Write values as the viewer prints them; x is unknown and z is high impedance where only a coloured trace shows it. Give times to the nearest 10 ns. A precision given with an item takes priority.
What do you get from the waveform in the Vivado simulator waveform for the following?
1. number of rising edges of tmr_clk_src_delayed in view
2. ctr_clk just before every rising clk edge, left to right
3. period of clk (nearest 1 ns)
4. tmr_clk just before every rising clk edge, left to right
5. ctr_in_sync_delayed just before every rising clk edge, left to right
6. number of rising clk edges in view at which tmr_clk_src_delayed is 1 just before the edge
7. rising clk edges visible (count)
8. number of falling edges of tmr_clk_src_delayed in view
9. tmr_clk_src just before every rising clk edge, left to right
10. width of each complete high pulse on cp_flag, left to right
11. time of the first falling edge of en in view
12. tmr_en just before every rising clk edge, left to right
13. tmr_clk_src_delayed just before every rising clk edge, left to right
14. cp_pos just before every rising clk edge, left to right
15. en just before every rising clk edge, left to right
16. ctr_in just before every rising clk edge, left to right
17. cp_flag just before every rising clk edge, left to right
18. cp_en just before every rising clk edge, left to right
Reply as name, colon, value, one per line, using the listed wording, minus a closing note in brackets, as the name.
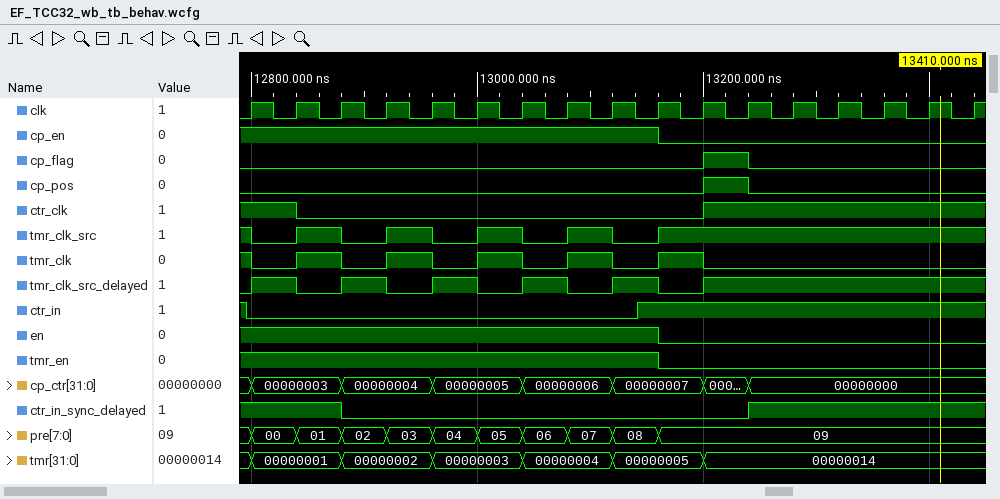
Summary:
number of rising edges of tmr_clk_src_delayed in view: 6
ctr_clk just before every rising clk edge, left to right: 1 1 0 0 0 0 0 0 0 0 0 1 1 1 1 1 1
period of clk: 40 ns
tmr_clk just before every rising clk edge, left to right: 1 0 1 0 1 0 1 0 1 0 1 0 0 0 0 0 0
ctr_in_sync_delayed just before every rising clk edge, left to right: 1 1 1 0 0 0 0 0 0 0 0 0 1 1 1 1 1
number of rising clk edges in view at which tmr_clk_src_delayed is 1 just before the edge: 11
rising clk edges visible: 17
number of falling edges of tmr_clk_src_delayed in view: 5
tmr_clk_src just before every rising clk edge, left to right: 1 0 1 0 1 0 1 0 1 0 1 1 1 1 1 1 1
width of each complete high pulse on cp_flag, left to right: 40 ns
time of the first falling edge of en in view: 13160 ns
tmr_en just before every rising clk edge, left to right: 1 1 1 1 1 1 1 1 1 1 0 0 0 0 0 0 0
tmr_clk_src_delayed just before every rising clk edge, left to right: 0 1 0 1 0 1 0 1 0 1 0 1 1 1 1 1 1
cp_pos just before every rising clk edge, left to right: 0 0 0 0 0 0 0 0 0 0 0 1 0 0 0 0 0
en just before every rising clk edge, left to right: 1 1 1 1 1 1 1 1 1 1 0 0 0 0 0 0 0
ctr_in just before every rising clk edge, left to right: 0 0 0 0 0 0 0 0 0 1 1 1 1 1 1 1 1
cp_flag just before every rising clk edge, left to right: 0 0 0 0 0 0 0 0 0 0 0 1 0 0 0 0 0
cp_en just before every rising clk edge, left to right: 1 1 1 1 1 1 1 1 1 1 0 0 0 0 0 0 0
